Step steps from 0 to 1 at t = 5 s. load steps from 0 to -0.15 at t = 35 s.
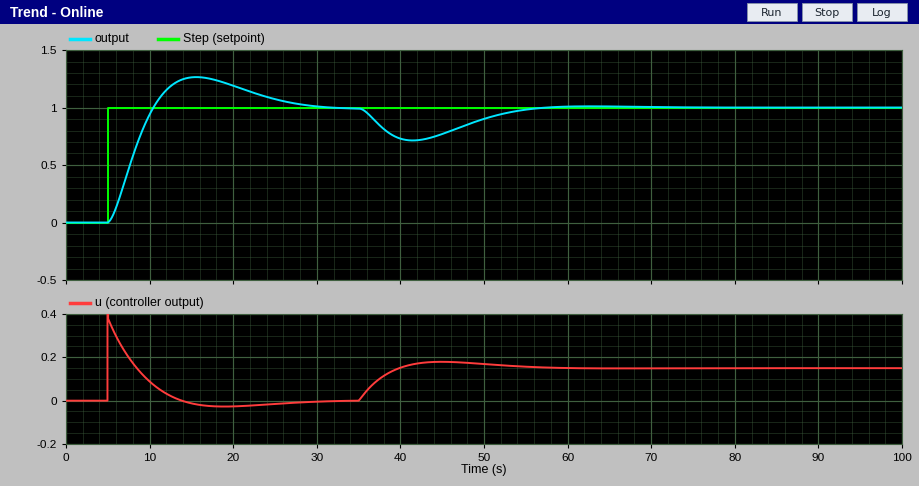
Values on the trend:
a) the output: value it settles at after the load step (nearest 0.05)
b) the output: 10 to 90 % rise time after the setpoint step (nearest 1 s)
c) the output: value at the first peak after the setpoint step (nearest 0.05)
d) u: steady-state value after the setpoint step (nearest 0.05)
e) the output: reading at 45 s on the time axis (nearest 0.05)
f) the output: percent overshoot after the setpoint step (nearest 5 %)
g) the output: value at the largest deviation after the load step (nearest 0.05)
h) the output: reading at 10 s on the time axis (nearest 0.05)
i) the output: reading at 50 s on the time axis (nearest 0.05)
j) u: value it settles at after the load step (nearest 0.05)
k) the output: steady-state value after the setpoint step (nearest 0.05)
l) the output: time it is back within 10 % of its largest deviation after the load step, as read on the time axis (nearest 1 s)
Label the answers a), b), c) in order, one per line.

a) 1.00
b) 4 s
c) 1.25
d) 0.00
e) 0.75
f) 25 %
g) 0.70
h) 0.95
i) 0.90
j) 0.15
k) 1.00
l) 54 s
